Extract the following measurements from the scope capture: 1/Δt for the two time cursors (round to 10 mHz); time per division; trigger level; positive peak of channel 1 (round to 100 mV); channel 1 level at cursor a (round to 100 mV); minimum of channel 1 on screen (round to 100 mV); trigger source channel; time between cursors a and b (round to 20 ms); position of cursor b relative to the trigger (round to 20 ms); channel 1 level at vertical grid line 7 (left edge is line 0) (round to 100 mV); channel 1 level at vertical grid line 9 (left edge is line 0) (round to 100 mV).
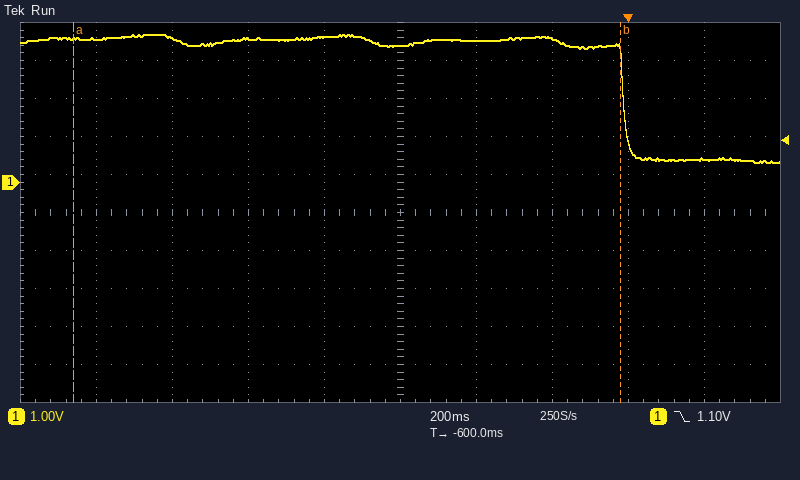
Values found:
690 mHz
200 ms
1.10 V
3.9 V
3.8 V
500 mV
channel 1
1.44 s
-20 ms
3.8 V
600 mV
